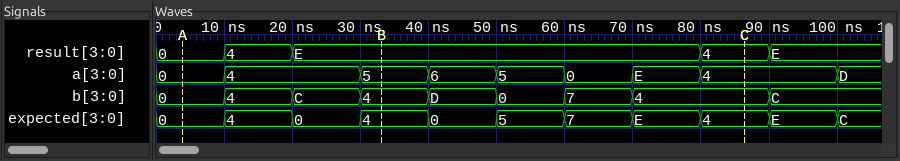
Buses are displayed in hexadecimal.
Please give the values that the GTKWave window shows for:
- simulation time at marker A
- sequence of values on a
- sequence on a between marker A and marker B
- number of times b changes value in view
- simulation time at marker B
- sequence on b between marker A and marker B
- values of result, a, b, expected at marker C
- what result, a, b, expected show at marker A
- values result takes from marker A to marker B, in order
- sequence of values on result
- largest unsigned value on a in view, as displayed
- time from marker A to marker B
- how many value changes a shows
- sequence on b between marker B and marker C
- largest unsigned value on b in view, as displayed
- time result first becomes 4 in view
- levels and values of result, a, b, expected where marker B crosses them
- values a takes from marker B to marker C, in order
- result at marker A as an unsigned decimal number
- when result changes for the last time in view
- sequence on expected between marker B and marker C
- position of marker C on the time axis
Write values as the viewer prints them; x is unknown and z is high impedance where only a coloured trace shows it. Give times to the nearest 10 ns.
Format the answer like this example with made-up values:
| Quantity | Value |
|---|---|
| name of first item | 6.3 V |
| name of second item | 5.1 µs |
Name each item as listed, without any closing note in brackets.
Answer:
| Quantity | Value |
|---|---|
| simulation time at marker A | 0 ns |
| sequence of values on a | 0, 4, 5, 6, 5, 0, E, 4, D |
| sequence on a between marker A and marker B | 0, 4, 5 |
| number of times b changes value in view | 8 |
| simulation time at marker B | 30 ns |
| sequence on b between marker A and marker B | 0, 4, C, 4 |
| values of result, a, b, expected at marker C | result=4, a=4, b=4, expected=4 |
| what result, a, b, expected show at marker A | result=0, a=0, b=0, expected=0 |
| values result takes from marker A to marker B, in order | 0, 4, E |
| sequence of values on result | 0, 4, E, 4, E |
| largest unsigned value on a in view, as displayed | E |
| time from marker A to marker B | 30 ns |
| how many value changes a shows | 8 |
| sequence on b between marker B and marker C | 4, D, 0, 7, 4 |
| largest unsigned value on b in view, as displayed | D |
| time result first becomes 4 in view | 10 ns |
| levels and values of result, a, b, expected where marker B crosses them | result=E, a=5, b=4, expected=4 |
| values a takes from marker B to marker C, in order | 5, 6, 5, 0, E, 4 |
| result at marker A as an unsigned decimal number | 0 |
| when result changes for the last time in view | 90 ns |
| sequence on expected between marker B and marker C | 4, 0, 5, 7, E, 4 |
| position of marker C on the time axis | 90 ns |
